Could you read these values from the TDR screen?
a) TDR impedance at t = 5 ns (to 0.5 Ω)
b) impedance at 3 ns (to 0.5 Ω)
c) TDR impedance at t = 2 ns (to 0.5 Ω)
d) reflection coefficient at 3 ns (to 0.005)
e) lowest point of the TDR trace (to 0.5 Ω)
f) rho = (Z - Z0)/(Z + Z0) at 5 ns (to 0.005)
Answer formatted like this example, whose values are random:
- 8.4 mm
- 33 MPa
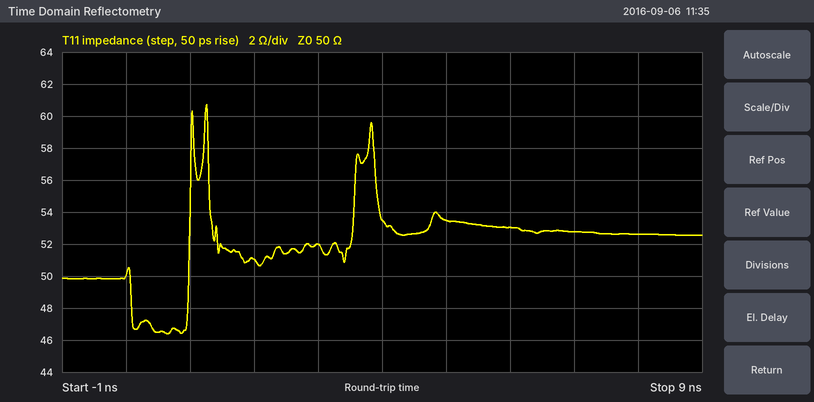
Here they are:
- 53.5 Ω
- 52.0 Ω
- 51.0 Ω
- +0.020
- 46.5 Ω
- +0.035
